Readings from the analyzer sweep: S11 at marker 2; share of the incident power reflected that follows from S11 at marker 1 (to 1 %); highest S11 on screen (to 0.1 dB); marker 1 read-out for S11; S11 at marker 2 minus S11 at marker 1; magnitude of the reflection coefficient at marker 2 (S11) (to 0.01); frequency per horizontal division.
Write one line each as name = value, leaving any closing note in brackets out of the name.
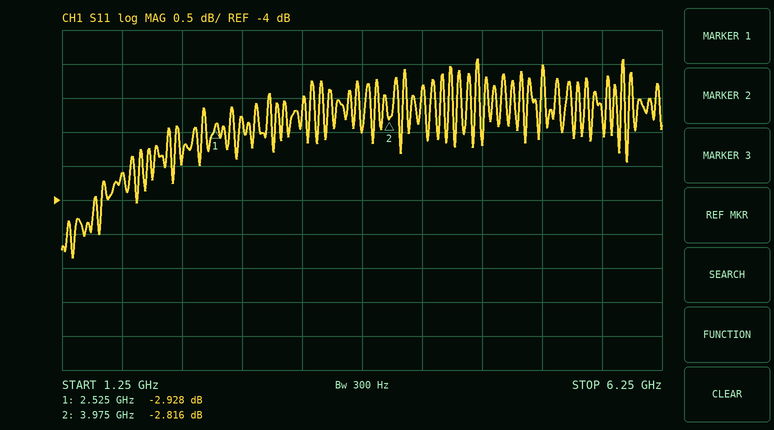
S11 at marker 2 = -2.816 dB
share of the incident power reflected that follows from S11 at marker 1 = 51 %
highest S11 on screen = -1.9 dB
marker 1 read-out for S11 = -2.928 dB
S11 at marker 2 minus S11 at marker 1 = 0.112 dB
magnitude of the reflection coefficient at marker 2 (S11) = 0.72
frequency per horizontal division = 500 MHz
